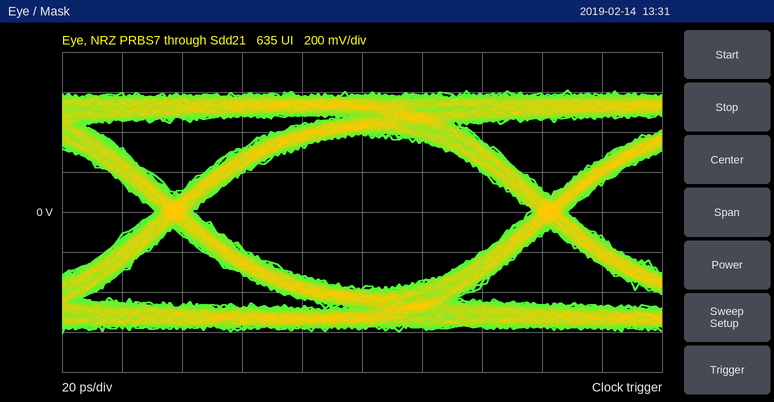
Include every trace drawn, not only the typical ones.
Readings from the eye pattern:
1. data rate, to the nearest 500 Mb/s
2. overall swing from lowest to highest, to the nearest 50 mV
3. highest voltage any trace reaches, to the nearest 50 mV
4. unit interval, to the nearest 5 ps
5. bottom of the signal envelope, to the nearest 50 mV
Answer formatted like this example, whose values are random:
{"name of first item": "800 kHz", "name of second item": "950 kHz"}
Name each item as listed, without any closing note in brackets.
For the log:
{"data rate, to the nearest 500 Mb/s": "8.0 Gb/s", "overall swing from lowest to highest, to the nearest 50 mV": "1.20 V", "highest voltage any trace reaches, to the nearest 50 mV": "600 mV", "unit interval, to the nearest 5 ps": "125 ps", "bottom of the signal envelope, to the nearest 50 mV": "-600 mV"}
